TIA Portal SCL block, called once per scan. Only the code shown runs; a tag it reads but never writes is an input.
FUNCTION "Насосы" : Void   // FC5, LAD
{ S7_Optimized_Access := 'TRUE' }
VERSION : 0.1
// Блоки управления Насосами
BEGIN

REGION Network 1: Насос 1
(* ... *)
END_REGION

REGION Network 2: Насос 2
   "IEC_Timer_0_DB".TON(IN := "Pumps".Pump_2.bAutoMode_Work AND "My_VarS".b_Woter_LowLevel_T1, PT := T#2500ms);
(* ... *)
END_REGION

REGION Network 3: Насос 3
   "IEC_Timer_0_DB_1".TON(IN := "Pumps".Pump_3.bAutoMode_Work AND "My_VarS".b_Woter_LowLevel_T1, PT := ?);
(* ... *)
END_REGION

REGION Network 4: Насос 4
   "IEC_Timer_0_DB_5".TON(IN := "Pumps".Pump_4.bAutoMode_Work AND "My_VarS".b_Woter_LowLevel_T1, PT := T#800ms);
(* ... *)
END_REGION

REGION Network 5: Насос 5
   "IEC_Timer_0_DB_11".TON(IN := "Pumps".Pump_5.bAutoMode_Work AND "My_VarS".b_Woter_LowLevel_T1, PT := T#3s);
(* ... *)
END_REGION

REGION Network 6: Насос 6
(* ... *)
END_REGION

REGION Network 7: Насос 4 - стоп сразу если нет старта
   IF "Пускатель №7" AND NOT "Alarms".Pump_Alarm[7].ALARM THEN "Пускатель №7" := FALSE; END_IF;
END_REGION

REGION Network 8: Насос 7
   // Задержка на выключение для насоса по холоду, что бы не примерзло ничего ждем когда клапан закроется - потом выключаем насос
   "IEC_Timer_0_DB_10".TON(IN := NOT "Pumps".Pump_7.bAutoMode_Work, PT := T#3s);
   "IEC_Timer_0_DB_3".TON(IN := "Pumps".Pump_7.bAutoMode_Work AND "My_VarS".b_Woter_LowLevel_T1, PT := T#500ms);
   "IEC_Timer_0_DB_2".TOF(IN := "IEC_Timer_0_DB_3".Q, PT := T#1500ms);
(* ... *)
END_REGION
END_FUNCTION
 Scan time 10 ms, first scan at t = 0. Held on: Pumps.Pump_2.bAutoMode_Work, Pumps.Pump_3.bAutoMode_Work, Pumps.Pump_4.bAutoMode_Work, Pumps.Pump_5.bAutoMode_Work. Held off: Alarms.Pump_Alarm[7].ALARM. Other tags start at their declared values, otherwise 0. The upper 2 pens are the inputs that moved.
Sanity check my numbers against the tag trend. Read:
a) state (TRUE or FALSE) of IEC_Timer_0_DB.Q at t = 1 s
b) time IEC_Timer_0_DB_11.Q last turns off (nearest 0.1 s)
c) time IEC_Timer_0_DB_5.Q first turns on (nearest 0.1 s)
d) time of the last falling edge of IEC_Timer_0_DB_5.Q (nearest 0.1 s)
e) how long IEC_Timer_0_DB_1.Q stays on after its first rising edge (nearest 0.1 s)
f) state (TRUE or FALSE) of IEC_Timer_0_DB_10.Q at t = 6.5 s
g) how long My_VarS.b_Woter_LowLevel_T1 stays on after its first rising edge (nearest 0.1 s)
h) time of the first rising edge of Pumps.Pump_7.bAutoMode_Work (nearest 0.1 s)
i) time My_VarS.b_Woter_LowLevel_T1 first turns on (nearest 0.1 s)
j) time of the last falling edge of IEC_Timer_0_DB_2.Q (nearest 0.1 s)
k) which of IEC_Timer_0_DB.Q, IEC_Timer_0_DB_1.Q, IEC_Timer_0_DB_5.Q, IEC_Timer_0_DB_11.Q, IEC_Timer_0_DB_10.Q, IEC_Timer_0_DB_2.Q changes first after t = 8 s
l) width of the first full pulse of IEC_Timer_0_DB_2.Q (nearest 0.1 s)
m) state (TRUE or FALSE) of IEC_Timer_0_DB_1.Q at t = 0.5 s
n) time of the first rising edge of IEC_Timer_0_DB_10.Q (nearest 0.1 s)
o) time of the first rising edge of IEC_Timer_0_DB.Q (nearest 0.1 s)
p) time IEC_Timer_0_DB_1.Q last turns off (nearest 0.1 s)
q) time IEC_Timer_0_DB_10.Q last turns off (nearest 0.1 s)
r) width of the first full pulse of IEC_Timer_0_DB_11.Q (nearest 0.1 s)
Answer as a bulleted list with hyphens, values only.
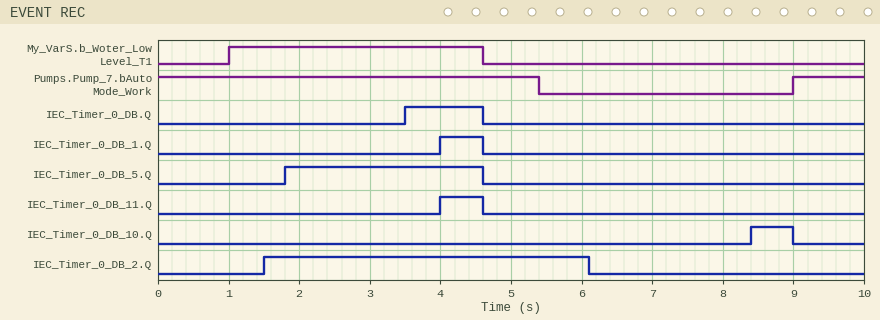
- FALSE
- 4.6 s
- 1.8 s
- 4.6 s
- 0.6 s
- FALSE
- 3.6 s
- 9.0 s
- 1.0 s
- 6.1 s
- IEC_Timer_0_DB_10.Q
- 4.6 s
- FALSE
- 8.4 s
- 3.5 s
- 4.6 s
- 9.0 s
- 0.6 s
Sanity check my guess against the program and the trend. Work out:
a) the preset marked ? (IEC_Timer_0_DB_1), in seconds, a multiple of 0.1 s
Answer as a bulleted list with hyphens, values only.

- 3.0 s
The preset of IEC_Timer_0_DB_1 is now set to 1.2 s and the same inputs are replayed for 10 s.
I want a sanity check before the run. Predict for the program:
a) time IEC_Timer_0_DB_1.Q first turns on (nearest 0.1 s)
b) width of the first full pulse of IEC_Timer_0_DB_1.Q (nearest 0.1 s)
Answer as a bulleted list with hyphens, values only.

- 2.2 s
- 2.4 s
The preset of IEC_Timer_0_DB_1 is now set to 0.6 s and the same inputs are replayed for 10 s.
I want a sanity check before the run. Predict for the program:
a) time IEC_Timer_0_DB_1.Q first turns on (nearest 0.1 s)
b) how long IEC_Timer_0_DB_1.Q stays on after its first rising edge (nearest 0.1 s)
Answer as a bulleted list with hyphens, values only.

- 1.6 s
- 3.0 s
